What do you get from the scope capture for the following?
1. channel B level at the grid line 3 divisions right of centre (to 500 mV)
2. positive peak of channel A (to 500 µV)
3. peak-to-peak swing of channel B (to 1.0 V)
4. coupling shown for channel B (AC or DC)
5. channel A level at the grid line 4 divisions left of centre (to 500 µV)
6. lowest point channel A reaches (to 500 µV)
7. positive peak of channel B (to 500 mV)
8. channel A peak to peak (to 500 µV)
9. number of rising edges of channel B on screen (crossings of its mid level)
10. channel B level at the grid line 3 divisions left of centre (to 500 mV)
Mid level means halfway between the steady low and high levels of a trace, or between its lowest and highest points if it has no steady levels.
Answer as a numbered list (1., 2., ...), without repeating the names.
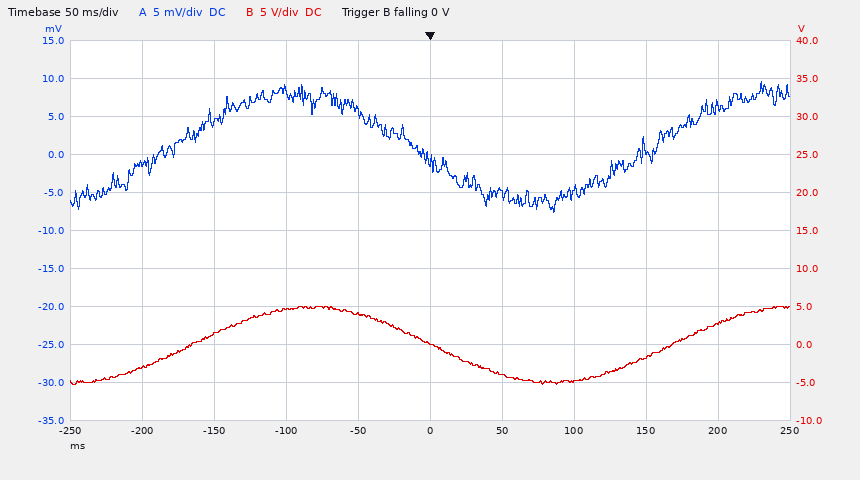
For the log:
1. -1.5 V
2. 9.5 mV
3. 10.0 V
4. DC
5. -1.0 mV
6. -7.5 mV
7. 5.0 V
8. 17.0 mV
9. 2
10. 1.5 V
